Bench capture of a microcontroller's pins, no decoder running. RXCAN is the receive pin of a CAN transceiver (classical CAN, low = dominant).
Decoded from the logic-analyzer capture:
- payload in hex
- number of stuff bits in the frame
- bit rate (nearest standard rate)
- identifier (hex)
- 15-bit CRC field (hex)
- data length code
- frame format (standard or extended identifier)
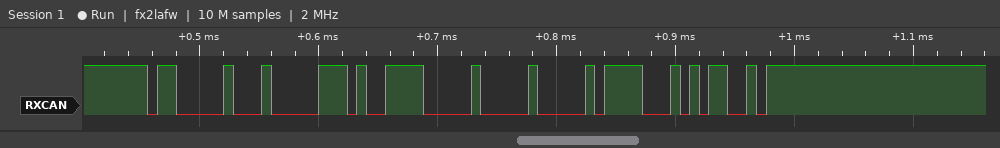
4F 00 00
5
125 kbit/s
0x601
0x78AC
3
standard
